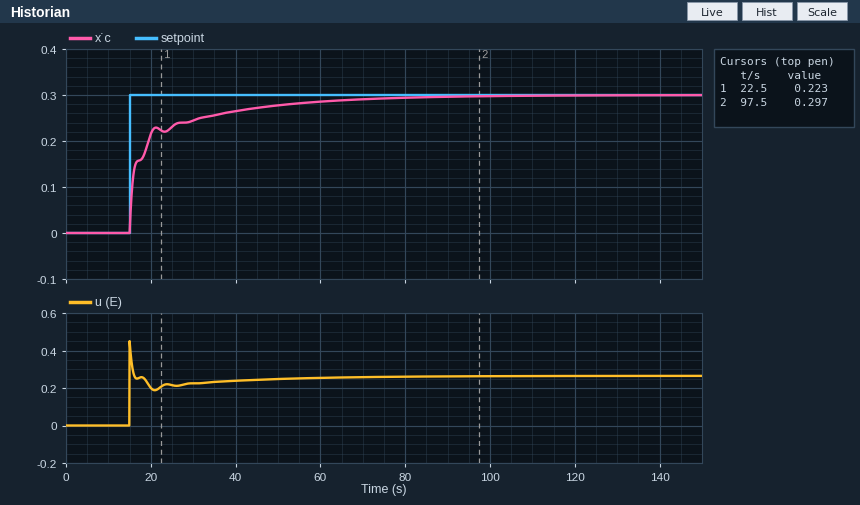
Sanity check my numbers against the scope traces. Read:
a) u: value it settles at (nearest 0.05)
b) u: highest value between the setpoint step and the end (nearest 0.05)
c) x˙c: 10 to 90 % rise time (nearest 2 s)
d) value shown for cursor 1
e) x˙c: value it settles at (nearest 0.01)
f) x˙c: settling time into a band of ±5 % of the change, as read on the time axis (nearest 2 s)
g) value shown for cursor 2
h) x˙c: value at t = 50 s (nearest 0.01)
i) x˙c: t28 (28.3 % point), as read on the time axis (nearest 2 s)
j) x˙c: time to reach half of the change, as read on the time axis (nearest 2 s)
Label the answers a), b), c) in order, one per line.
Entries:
a) 0.25
b) 0.45
c) 28 s
d) 0.223
e) 0.30
f) 60 s
g) 0.297
h) 0.28
i) 16 s
j) 16 s
